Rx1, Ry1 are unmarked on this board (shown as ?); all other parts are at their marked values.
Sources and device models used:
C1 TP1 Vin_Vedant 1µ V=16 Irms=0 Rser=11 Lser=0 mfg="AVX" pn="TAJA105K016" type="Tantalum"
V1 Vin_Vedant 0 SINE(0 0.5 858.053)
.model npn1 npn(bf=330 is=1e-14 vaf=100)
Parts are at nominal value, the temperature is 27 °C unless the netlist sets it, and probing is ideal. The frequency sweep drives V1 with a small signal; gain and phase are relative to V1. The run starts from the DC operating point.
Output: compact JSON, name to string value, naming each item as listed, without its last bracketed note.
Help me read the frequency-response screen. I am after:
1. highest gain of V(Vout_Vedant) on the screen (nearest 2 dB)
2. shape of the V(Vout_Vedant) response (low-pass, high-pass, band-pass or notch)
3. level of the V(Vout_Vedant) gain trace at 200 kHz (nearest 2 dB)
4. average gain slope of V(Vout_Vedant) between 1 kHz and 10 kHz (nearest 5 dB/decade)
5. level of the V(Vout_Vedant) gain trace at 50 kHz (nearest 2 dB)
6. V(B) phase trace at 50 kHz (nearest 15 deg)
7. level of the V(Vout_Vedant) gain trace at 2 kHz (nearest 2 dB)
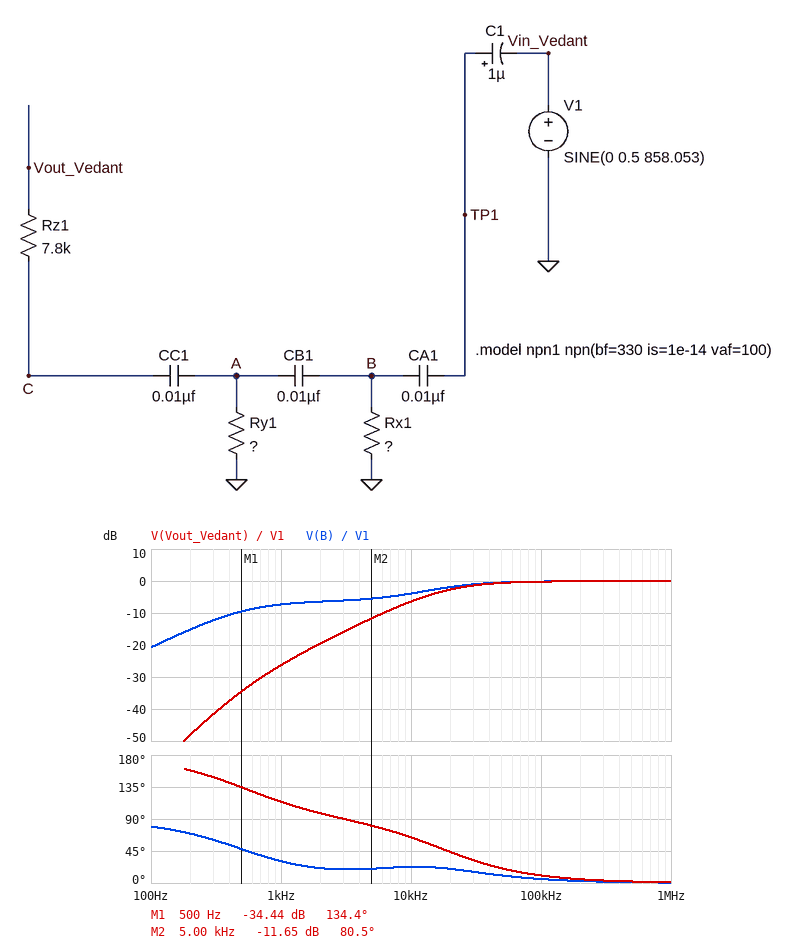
{"highest gain of V(Vout_Vedant) on the screen": "0 dB", "shape of the V(Vout_Vedant) response": "high-pass", "level of the V(Vout_Vedant) gain trace at 200 kHz": "0 dB", "average gain slope of V(Vout_Vedant) between 1 kHz and 10 kHz": "20 dB/decade", "level of the V(Vout_Vedant) gain trace at 50 kHz": "0 dB", "V(B) phase trace at 50 kHz": "15 deg", "level of the V(Vout_Vedant) gain trace at 2 kHz": "-20 dB"}
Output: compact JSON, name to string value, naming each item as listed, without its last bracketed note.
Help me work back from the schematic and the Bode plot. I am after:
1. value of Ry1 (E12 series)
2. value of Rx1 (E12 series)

{"value of Ry1": "1.8 kΩ", "value of Rx1": "15 kΩ"}
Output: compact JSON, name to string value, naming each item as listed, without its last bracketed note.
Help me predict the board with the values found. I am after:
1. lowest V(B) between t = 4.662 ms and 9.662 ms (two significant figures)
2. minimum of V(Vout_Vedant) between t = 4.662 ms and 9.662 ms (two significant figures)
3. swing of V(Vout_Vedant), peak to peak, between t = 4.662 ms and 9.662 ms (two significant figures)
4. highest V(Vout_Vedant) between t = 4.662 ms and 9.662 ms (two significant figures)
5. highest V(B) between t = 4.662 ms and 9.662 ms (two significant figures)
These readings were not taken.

{"lowest V(B) between t = 4.662 ms and 9.662 ms": "-210 mV", "minimum of V(Vout_Vedant) between t = 4.662 ms and 9.662 ms": "-20 mV", "swing of V(Vout_Vedant), peak to peak, between t = 4.662 ms and 9.662 ms": "40 mV", "highest V(Vout_Vedant) between t = 4.662 ms and 9.662 ms": "20 mV", "highest V(B) between t = 4.662 ms and 9.662 ms": "210 mV"}
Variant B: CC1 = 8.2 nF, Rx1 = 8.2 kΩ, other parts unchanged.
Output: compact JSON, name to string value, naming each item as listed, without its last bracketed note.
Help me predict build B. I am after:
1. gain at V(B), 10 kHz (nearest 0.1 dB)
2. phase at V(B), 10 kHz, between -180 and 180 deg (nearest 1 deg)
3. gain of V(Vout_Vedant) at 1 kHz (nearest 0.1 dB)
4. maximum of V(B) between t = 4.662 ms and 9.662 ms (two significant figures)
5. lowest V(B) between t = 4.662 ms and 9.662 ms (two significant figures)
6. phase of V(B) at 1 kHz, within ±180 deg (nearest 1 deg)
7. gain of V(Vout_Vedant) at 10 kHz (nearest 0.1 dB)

{"gain at V(B), 10 kHz": "-4.1 dB", "phase at V(B), 10 kHz, between -180 and 180 deg": "26 deg", "gain of V(Vout_Vedant) at 1 kHz": "-28.2 dB", "maximum of V(B) between t = 4.662 ms and 9.662 ms": "160 mV", "lowest V(B) between t = 4.662 ms and 9.662 ms": "-160 mV", "phase of V(B) at 1 kHz, within ±180 deg": "46 deg", "gain of V(Vout_Vedant) at 10 kHz": "-6.6 dB"}
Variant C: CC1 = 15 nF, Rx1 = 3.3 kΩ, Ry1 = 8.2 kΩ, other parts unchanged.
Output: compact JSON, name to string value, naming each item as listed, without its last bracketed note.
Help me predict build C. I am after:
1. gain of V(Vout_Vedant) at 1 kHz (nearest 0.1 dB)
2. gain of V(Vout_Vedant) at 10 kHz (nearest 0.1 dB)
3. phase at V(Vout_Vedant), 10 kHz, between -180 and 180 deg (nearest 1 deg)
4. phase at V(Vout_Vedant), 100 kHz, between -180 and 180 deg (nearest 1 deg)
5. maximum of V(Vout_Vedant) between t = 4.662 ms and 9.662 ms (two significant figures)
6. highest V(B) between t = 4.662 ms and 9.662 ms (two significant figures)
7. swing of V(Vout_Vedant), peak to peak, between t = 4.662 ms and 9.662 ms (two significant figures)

{"gain of V(Vout_Vedant) at 1 kHz": "-21.7 dB", "gain of V(Vout_Vedant) at 10 kHz": "-2.0 dB", "phase at V(Vout_Vedant), 10 kHz, between -180 and 180 deg": "44 deg", "phase at V(Vout_Vedant), 100 kHz, between -180 and 180 deg": "5 deg", "maximum of V(Vout_Vedant) between t = 4.662 ms and 9.662 ms": "32 mV", "highest V(B) between t = 4.662 ms and 9.662 ms": "79 mV", "swing of V(Vout_Vedant), peak to peak, between t = 4.662 ms and 9.662 ms": "64 mV"}
